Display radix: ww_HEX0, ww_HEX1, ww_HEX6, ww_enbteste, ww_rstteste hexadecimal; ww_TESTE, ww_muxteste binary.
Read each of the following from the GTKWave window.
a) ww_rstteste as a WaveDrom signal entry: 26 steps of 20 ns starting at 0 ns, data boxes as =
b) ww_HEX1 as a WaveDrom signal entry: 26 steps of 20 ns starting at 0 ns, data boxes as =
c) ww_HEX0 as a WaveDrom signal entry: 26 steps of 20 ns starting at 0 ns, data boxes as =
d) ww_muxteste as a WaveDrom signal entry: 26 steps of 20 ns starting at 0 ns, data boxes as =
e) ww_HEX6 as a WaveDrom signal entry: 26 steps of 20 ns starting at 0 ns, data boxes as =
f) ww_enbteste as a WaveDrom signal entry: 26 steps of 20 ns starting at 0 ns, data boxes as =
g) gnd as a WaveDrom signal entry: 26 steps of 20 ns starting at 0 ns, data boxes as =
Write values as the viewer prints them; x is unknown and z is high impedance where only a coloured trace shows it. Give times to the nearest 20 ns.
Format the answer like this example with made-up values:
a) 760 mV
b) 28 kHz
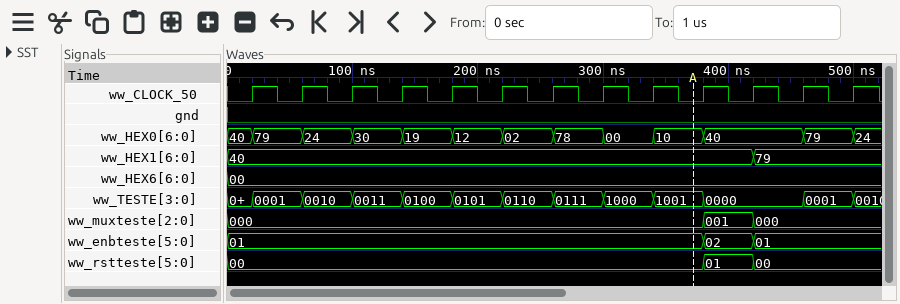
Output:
a) {name: 'ww_rstteste', wave: '=..................=.=....', data: '00 01 00'}
b) {name: 'ww_HEX1', wave: '=....................=....', data: '40 79'}
c) {name: 'ww_HEX0', wave: '==.=.=.=.=.=.=.=.=.=...=.=', data: '40 79 24 30 19 12 02 78 00 10 40 79 24'}
d) {name: 'ww_muxteste', wave: '=..................=.=....', data: '000 001 000'}
e) {name: 'ww_HEX6', wave: '=.........................', data: '00'}
f) {name: 'ww_enbteste', wave: '=..................=.=....', data: '01 02 01'}
g) {name: 'gnd', wave: '0.........................'}
